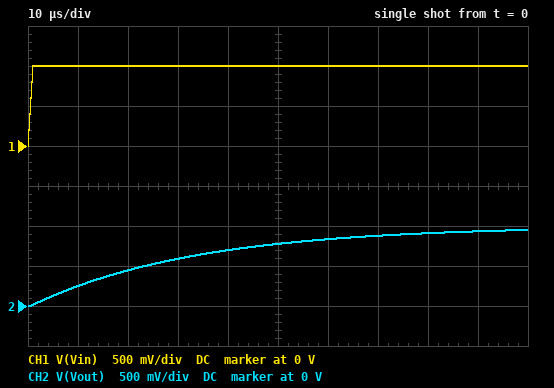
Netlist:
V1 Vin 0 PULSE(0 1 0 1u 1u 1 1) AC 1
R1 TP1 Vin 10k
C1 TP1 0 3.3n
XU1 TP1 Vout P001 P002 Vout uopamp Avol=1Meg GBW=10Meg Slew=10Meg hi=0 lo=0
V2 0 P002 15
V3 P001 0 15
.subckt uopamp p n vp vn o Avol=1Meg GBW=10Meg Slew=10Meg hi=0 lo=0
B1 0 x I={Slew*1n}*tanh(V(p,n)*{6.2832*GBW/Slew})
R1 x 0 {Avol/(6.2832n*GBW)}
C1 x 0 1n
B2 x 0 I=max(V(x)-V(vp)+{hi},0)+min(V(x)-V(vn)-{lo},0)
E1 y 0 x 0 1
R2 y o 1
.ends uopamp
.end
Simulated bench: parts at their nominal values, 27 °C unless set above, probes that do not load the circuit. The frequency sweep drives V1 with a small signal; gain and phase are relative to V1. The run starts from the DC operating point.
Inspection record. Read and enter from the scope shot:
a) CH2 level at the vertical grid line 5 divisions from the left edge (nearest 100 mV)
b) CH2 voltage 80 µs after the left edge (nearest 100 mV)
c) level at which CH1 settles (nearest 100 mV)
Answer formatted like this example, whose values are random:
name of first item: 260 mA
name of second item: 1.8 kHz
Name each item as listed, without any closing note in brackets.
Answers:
CH2 level at the vertical grid line 5 divisions from the left edge: 800 mV
CH2 voltage 80 µs after the left edge: 900 mV
level at which CH1 settles: 1.0 V
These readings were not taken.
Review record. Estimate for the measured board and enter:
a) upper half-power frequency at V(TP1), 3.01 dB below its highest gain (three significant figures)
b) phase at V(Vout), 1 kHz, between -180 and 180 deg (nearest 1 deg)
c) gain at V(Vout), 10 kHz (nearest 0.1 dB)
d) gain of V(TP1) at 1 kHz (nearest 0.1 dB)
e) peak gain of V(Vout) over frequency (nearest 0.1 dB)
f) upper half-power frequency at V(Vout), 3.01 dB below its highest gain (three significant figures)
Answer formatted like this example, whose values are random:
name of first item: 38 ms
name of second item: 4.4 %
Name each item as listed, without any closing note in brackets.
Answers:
upper half-power frequency at V(TP1), 3.01 dB below its highest gain: 4.82 kHz
phase at V(Vout), 1 kHz, between -180 and 180 deg: -12 deg
gain at V(Vout), 10 kHz: -7.2 dB
gain of V(TP1) at 1 kHz: -0.2 dB
peak gain of V(Vout) over frequency: 0 dB
upper half-power frequency at V(Vout), 3.01 dB below its highest gain: 4.82 kHz
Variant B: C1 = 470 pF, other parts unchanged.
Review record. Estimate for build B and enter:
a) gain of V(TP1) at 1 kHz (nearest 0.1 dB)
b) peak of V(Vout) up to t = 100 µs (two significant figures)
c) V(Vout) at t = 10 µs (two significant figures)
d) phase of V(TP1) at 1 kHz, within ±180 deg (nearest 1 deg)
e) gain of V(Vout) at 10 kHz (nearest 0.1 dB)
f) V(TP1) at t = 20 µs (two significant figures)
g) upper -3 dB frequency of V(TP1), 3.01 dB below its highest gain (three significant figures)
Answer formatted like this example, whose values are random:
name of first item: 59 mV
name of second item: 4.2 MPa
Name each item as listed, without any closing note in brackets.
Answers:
gain of V(TP1) at 1 kHz: 0 dB
peak of V(Vout) up to t = 100 µs: 1.0 V
V(Vout) at t = 10 µs: 870 mV
phase of V(TP1) at 1 kHz, within ±180 deg: -2 deg
gain of V(Vout) at 10 kHz: -0.4 dB
V(TP1) at t = 20 µs: 980 mV
upper -3 dB frequency of V(TP1), 3.01 dB below its highest gain: 33.9 kHz
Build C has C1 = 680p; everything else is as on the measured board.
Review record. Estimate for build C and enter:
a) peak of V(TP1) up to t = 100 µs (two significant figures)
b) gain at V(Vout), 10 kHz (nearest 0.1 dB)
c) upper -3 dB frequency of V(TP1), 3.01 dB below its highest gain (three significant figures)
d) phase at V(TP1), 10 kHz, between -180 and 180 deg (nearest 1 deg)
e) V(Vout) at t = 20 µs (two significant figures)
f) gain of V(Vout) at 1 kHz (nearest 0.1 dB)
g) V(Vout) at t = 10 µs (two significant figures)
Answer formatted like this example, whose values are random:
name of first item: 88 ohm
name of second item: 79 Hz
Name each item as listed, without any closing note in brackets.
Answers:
peak of V(TP1) up to t = 100 µs: 1.0 V
gain at V(Vout), 10 kHz: -0.7 dB
upper -3 dB frequency of V(TP1), 3.01 dB below its highest gain: 23.4 kHz
phase at V(TP1), 10 kHz, between -180 and 180 deg: -23 deg
V(Vout) at t = 20 µs: 940 mV
gain of V(Vout) at 1 kHz: 0 dB
V(Vout) at t = 10 µs: 750 mV
